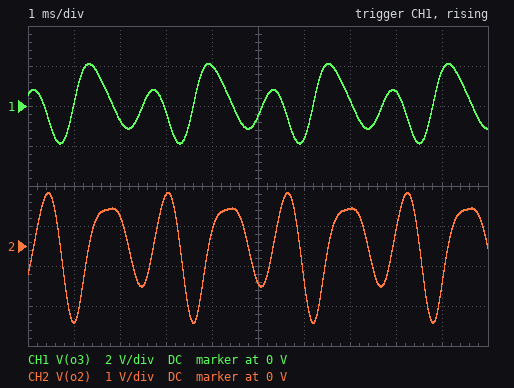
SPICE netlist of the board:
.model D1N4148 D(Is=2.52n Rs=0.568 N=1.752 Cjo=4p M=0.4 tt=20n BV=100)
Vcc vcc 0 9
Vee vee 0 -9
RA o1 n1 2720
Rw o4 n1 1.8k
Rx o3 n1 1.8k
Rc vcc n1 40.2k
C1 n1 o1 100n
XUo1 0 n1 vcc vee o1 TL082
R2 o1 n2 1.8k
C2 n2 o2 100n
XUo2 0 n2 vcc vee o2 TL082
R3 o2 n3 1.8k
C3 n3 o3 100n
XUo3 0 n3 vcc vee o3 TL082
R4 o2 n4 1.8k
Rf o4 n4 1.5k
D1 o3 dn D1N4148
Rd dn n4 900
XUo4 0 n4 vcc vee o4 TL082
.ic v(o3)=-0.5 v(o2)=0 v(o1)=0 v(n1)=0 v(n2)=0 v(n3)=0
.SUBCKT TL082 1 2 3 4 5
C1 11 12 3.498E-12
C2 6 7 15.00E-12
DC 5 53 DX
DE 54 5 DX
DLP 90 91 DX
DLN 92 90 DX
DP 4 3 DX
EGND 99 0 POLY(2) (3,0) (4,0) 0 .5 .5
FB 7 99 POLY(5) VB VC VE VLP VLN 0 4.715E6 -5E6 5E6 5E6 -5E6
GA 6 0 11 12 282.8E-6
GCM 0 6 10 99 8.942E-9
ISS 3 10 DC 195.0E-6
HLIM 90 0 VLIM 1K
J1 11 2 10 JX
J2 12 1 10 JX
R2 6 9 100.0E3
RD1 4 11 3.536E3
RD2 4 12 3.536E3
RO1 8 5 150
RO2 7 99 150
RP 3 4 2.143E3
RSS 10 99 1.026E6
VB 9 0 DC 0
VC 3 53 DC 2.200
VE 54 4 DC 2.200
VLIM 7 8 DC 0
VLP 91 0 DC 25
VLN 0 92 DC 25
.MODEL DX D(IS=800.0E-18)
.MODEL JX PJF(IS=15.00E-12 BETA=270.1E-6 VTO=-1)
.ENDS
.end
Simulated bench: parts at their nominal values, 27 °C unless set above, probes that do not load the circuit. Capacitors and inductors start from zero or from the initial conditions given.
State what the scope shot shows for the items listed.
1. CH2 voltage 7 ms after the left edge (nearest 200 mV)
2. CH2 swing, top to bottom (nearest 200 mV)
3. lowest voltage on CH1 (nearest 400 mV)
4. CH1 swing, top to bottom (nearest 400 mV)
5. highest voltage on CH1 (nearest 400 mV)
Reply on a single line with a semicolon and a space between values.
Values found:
1.0 V; 3.2 V; -2.0 V; 4.0 V; 2.0 V
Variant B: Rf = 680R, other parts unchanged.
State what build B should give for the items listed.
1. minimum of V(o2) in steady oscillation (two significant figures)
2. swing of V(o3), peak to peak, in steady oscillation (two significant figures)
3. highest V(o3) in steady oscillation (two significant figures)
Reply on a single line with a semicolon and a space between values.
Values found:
-7.5 V; 15 V; 7.5 V
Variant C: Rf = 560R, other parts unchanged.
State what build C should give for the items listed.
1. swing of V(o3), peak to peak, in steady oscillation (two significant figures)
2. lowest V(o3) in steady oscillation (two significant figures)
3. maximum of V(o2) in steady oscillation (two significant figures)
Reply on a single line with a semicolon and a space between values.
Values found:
15 V; -7.5 V; 7.5 V
